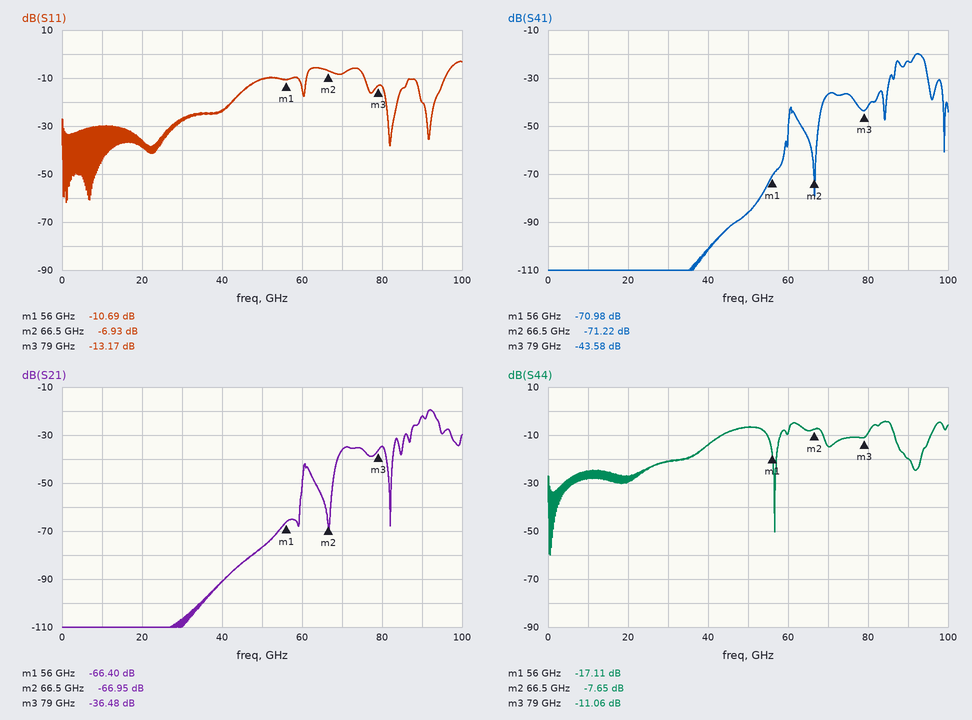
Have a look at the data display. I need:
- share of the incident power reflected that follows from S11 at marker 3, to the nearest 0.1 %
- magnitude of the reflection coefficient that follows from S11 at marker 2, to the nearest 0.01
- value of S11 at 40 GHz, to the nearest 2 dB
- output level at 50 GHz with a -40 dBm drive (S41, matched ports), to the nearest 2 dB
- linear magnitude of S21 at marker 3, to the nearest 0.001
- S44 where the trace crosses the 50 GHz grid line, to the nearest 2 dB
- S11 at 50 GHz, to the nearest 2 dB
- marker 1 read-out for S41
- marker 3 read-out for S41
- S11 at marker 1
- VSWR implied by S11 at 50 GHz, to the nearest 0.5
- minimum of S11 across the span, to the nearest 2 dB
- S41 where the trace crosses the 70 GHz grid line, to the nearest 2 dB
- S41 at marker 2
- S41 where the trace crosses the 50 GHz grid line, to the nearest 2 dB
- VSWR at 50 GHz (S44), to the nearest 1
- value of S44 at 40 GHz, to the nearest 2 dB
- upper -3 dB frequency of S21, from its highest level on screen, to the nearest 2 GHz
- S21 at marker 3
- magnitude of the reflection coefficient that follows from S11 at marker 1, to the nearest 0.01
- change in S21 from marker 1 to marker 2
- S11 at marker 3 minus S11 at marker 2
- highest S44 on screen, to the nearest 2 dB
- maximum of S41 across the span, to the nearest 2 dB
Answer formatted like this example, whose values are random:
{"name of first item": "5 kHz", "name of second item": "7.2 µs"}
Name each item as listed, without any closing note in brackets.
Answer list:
{"share of the incident power reflected that follows from S11 at marker 3, to the nearest 0.1 %": "4.8 %", "magnitude of the reflection coefficient that follows from S11 at marker 2, to the nearest 0.01": "0.45", "value of S11 at 40 GHz, to the nearest 2 dB": "-24 dB", "output level at 50 GHz with a -40 dBm drive (S41, matched ports), to the nearest 2 dB": "-126 dBm", "linear magnitude of S21 at marker 3, to the nearest 0.001": "0.015", "S44 where the trace crosses the 50 GHz grid line, to the nearest 2 dB": "-6 dB", "S11 at 50 GHz, to the nearest 2 dB": "-10 dB", "marker 1 read-out for S41": "-70.98 dB", "marker 3 read-out for S41": "-43.58 dB", "S11 at marker 1": "-10.69 dB", "VSWR implied by S11 at 50 GHz, to the nearest 0.5": "2.0", "minimum of S11 across the span, to the nearest 2 dB": "-62 dB", "S41 where the trace crosses the 70 GHz grid line, to the nearest 2 dB": "-36 dB", "S41 at marker 2": "-71.22 dB", "S41 where the trace crosses the 50 GHz grid line, to the nearest 2 dB": "-86 dB", "VSWR at 50 GHz (S44), to the nearest 1": "3", "value of S44 at 40 GHz, to the nearest 2 dB": "-14 dB", "upper -3 dB frequency of S21, from its highest level on screen, to the nearest 2 GHz": "94 GHz", "S21 at marker 3": "-36.48 dB", "magnitude of the reflection coefficient that follows from S11 at marker 1, to the nearest 0.01": "0.29", "change in S21 from marker 1 to marker 2": "-0.55 dB", "S11 at marker 3 minus S11 at marker 2": "-6.24 dB", "highest S44 on screen, to the nearest 2 dB": "-4 dB", "maximum of S41 across the span, to the nearest 2 dB": "-20 dB"}
